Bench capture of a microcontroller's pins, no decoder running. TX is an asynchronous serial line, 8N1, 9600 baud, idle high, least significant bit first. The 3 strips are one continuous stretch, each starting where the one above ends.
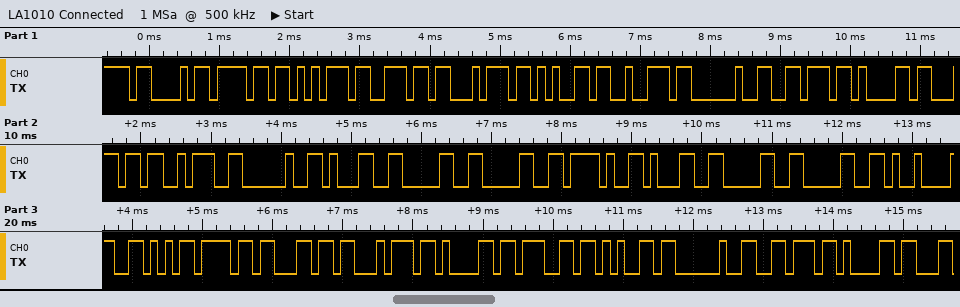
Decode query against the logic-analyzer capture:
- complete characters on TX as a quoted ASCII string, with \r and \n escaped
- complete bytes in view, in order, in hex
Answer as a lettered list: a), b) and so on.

a) "Counter val: 100/100\tVoltage va"
b) 43 6F 75 6E 74 65 72 20 76 61 6C 3A 20 31 30 30 2F 31 30 30 09 56 6F 6C 74 61 67 65 20 76 61
